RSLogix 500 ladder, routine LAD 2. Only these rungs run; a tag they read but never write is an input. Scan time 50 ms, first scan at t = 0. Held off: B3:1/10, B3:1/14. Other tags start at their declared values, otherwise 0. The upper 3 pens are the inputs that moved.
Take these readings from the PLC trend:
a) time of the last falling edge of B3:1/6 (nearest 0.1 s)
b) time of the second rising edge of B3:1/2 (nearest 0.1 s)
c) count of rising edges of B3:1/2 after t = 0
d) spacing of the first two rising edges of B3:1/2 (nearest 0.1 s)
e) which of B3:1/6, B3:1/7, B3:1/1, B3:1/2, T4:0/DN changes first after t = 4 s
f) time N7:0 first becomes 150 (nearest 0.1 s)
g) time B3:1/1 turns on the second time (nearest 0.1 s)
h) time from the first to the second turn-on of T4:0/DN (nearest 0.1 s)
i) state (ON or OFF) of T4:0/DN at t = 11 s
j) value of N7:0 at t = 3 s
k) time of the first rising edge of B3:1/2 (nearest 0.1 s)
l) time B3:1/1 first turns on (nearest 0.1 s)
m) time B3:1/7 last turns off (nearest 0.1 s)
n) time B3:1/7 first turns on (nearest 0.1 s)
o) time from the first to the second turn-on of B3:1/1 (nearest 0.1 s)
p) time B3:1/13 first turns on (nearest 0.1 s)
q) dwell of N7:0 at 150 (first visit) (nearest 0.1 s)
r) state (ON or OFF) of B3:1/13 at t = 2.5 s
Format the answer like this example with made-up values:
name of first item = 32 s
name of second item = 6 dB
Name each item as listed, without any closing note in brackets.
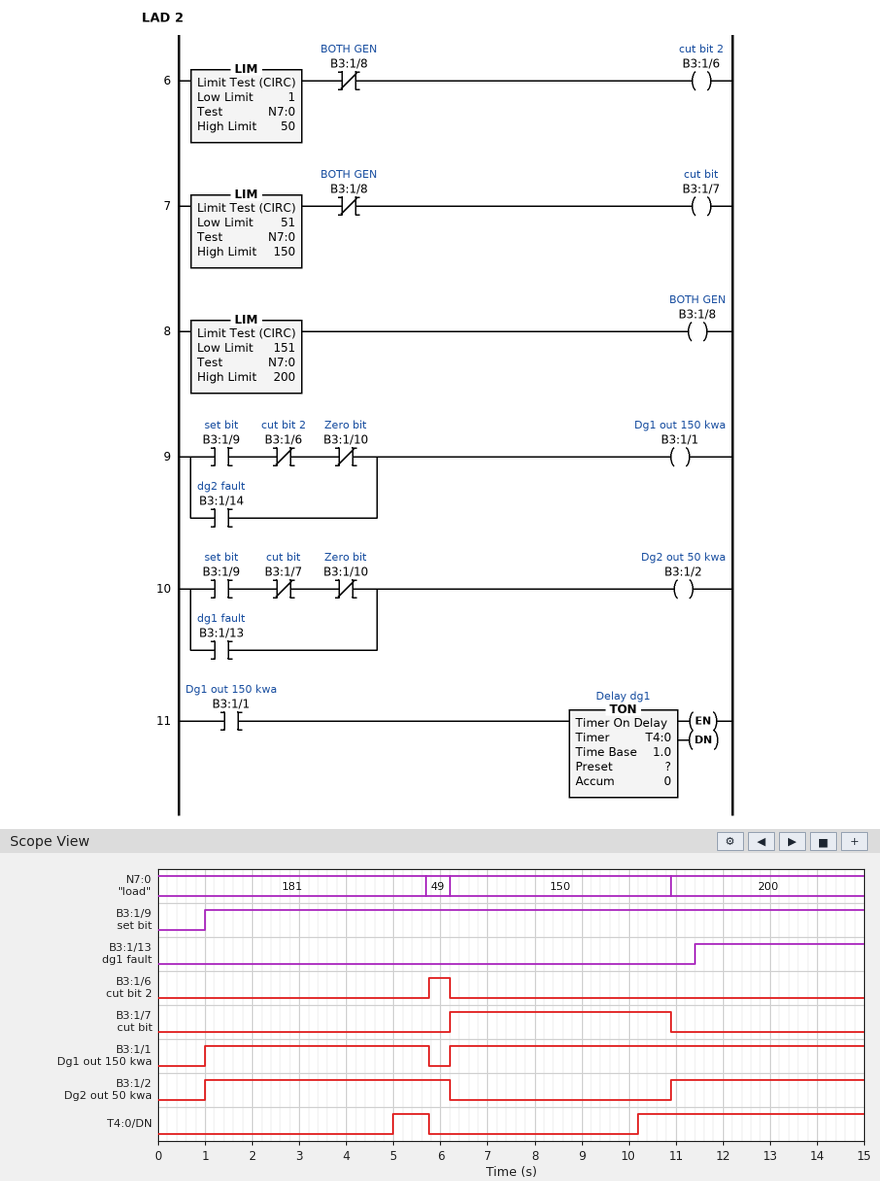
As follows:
time of the last falling edge of B3:1/6 = 6.2 s
time of the second rising edge of B3:1/2 = 10.9 s
count of rising edges of B3:1/2 after t = 0 = 2
spacing of the first two rising edges of B3:1/2 = 9.9 s
which of B3:1/6, B3:1/7, B3:1/1, B3:1/2, T4:0/DN changes first after t = 4 s = T4:0/DN
time N7:0 first becomes 150 = 6.2 s
time B3:1/1 turns on the second time = 6.2 s
time from the first to the second turn-on of T4:0/DN = 5.2 s
state (ON or OFF) of T4:0/DN at t = 11 s = ON
value of N7:0 at t = 3 s = 181
time of the first rising edge of B3:1/2 = 1.0 s
time B3:1/1 first turns on = 1.0 s
time B3:1/7 last turns off = 10.9 s
time B3:1/7 first turns on = 6.2 s
time from the first to the second turn-on of B3:1/1 = 5.2 s
time B3:1/13 first turns on = 11.4 s
dwell of N7:0 at 150 (first visit) = 4.7 s
state (ON or OFF) of B3:1/13 at t = 2.5 s = OFF
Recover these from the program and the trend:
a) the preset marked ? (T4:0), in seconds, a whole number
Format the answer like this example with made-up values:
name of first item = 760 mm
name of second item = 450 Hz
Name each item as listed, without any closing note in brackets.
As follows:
the preset marked ? (T4:0), in seconds, a whole number = 4 s
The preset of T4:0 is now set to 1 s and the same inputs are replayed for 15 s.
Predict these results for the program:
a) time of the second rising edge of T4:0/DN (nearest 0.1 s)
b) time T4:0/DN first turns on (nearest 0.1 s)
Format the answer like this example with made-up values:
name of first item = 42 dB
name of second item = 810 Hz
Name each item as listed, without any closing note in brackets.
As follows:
time of the second rising edge of T4:0/DN = 7.2 s
time T4:0/DN first turns on = 2.0 s
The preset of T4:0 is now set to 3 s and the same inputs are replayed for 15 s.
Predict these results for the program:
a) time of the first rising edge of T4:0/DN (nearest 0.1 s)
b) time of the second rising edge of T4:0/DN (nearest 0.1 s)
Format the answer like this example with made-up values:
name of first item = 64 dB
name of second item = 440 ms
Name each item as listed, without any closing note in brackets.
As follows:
time of the first rising edge of T4:0/DN = 4.0 s
time of the second rising edge of T4:0/DN = 9.2 s
